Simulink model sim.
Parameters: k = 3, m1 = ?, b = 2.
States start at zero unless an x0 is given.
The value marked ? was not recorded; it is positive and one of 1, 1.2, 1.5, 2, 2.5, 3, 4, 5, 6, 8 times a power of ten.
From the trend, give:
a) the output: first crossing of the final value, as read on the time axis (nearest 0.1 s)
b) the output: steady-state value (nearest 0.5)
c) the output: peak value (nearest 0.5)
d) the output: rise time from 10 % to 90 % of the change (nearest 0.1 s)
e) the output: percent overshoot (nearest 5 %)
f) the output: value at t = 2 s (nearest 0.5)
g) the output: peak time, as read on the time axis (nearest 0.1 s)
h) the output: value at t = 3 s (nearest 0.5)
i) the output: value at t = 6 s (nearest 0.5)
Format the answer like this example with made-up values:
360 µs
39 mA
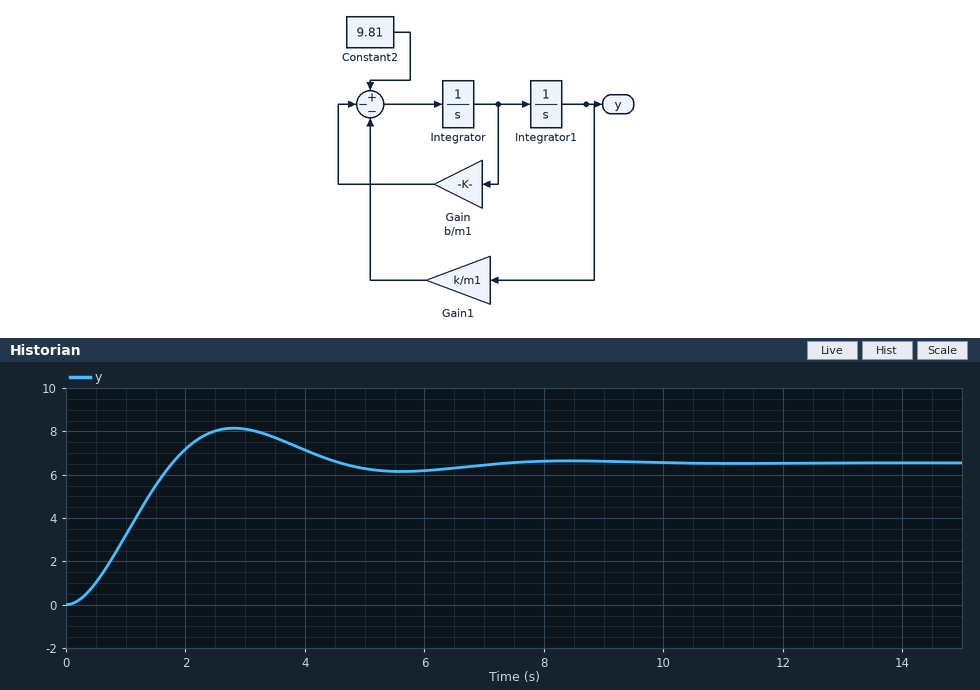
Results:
1.8 s
6.5
8.0
1.2 s
25 %
7.0
2.8 s
8.0
6.0
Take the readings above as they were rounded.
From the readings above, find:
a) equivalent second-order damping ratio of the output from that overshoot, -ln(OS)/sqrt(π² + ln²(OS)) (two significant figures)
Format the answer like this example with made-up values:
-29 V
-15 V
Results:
0.40
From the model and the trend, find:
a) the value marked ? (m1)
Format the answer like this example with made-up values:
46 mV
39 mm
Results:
2
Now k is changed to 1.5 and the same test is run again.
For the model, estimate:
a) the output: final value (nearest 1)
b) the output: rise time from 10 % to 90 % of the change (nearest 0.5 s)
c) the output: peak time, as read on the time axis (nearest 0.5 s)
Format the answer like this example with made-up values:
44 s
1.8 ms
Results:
13
2.0 s
4.5 s
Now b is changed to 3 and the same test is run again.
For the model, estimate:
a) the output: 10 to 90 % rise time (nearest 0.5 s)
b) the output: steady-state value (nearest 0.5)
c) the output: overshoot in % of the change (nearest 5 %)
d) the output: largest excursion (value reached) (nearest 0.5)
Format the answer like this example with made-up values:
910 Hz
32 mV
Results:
1.5 s
6.5
10 %
7.0
